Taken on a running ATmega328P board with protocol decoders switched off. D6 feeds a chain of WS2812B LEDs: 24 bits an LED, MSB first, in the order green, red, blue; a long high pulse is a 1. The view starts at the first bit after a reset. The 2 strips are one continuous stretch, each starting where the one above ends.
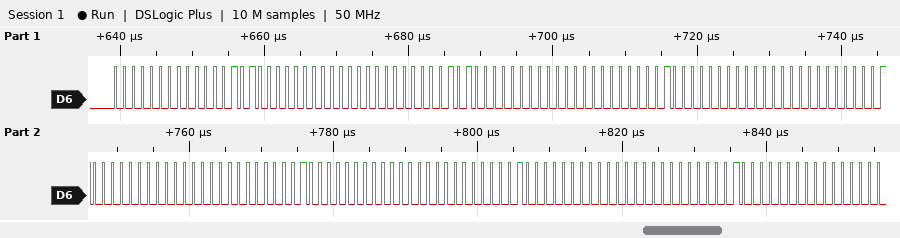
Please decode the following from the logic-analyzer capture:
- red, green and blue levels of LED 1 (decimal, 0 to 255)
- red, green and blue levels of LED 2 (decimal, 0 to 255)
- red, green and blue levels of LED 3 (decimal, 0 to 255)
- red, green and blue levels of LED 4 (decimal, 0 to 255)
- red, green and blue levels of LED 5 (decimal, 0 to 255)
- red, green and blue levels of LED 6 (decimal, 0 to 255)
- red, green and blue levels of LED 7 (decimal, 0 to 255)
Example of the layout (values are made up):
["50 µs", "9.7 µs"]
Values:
["5, 0, 0", "5, 0, 0", "4, 0, 0", "4, 0, 0", "4, 0, 0", "4, 0, 0", "4, 0, 0"]
